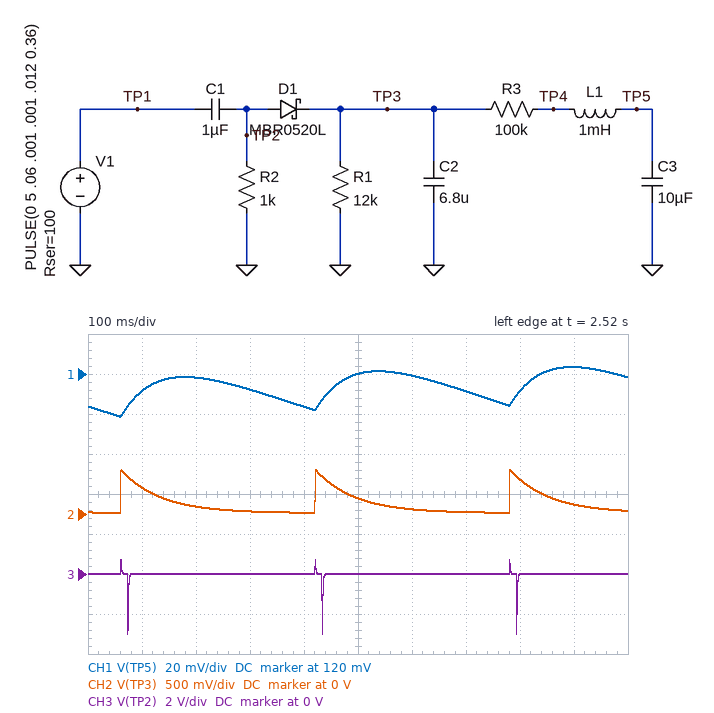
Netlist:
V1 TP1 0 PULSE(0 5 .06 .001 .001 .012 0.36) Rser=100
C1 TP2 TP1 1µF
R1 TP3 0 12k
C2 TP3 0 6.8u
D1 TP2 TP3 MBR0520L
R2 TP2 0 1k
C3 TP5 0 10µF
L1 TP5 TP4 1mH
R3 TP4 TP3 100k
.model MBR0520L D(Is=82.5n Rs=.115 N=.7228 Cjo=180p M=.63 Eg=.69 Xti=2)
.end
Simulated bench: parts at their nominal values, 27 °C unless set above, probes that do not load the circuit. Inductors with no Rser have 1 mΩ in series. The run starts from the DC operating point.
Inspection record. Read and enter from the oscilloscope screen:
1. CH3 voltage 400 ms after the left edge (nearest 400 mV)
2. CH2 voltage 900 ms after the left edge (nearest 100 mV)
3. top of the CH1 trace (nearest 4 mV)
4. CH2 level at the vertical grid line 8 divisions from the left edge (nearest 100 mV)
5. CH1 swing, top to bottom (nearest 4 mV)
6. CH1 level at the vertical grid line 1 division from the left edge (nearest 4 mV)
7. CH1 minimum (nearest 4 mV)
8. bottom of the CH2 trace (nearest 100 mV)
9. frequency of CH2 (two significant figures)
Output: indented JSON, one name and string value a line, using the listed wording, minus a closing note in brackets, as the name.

{
  "CH3 voltage 400 ms after the left edge": "0 V",
  "CH2 voltage 900 ms after the left edge": "100 mV",
  "top of the CH1 trace": "124 mV",
  "CH2 level at the vertical grid line 8 divisions from the left edge": "400 mV",
  "CH1 swing, top to bottom": "24 mV",
  "CH1 level at the vertical grid line 1 division from the left edge": "112 mV",
  "CH1 minimum": "100 mV",
  "bottom of the CH2 trace": "0 V",
  "frequency of CH2": "2.8 Hz"
}
